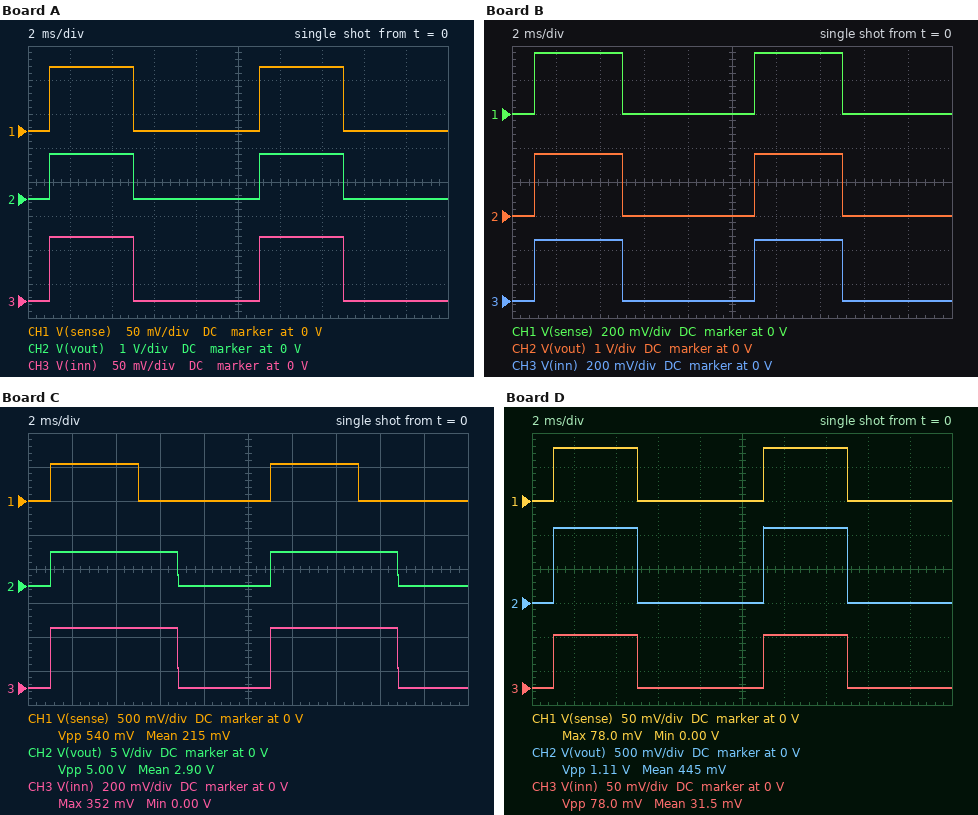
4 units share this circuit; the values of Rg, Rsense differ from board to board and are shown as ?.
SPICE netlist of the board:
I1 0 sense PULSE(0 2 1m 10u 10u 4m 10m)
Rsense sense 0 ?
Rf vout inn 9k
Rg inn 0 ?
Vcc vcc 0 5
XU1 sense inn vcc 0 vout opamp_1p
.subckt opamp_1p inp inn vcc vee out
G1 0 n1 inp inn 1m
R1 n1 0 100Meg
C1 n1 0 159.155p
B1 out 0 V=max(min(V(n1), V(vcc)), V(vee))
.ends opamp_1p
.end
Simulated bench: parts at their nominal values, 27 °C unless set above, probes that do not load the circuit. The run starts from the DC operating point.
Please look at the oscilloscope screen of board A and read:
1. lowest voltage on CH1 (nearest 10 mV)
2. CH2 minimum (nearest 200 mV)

0 V
0 V
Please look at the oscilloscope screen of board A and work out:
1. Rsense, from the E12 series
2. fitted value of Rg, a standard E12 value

0.047 Ω
680 Ω
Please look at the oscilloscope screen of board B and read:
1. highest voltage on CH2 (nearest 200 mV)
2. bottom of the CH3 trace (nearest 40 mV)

1.8 V
0 V
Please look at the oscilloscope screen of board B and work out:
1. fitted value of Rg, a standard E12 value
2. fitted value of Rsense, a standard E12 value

2.2 kΩ
0.18 Ω
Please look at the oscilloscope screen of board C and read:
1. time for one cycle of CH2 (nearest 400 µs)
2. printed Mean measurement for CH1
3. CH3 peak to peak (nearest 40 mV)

10.0 ms
215 mV
360 mV
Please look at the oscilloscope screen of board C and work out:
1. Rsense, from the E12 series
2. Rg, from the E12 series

0.27 Ω
680 Ω
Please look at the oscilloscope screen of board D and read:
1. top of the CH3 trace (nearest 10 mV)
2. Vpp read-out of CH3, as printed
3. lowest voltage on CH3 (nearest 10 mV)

80 mV
78.0 mV
0 V
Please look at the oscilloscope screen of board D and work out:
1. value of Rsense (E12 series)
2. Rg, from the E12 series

0.039 Ω
680 Ω
